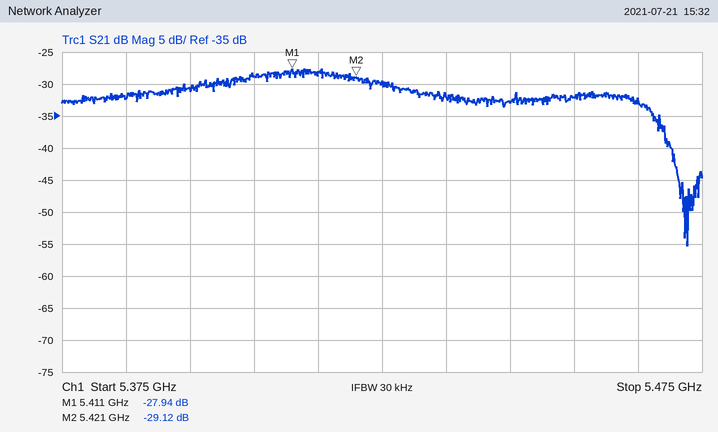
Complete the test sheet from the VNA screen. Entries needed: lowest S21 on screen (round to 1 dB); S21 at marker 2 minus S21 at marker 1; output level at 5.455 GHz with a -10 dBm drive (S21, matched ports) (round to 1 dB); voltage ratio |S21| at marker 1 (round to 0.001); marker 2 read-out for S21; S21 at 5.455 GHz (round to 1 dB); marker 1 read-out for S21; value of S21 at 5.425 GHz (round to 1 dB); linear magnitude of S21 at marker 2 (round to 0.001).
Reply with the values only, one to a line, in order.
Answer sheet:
-55 dB
-1.18 dB
-42 dBm
0.040
-29.12 dB
-32 dB
-27.94 dB
-30 dB
0.035
